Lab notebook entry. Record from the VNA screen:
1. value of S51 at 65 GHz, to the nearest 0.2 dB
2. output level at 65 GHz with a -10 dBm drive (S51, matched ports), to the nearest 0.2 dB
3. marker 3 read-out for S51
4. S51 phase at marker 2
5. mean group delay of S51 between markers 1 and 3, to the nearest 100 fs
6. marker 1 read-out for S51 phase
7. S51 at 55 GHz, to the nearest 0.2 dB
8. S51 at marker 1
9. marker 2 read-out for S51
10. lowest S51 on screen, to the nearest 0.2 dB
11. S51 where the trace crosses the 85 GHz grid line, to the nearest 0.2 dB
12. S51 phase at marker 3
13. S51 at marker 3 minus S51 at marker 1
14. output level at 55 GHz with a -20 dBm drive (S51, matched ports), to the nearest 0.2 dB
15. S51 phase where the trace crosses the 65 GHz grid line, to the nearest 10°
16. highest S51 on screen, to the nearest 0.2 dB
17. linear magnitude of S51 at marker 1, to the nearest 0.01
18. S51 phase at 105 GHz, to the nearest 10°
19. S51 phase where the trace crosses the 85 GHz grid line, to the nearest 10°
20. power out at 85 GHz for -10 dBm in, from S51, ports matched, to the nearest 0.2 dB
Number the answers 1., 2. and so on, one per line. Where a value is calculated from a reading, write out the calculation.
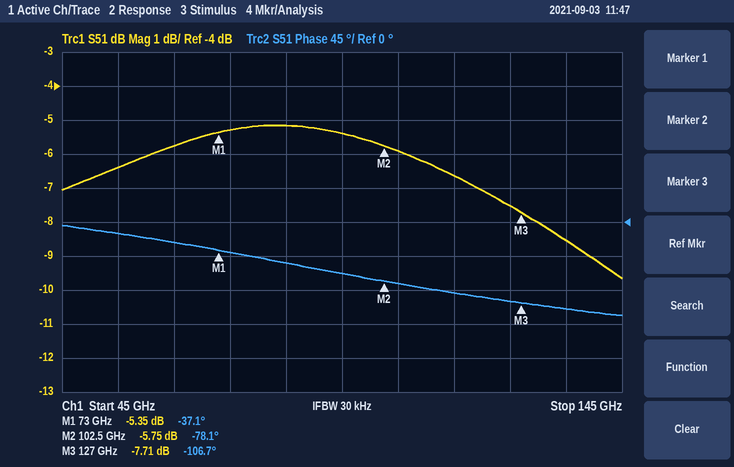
1. -5.8 dB
2. -10 dBm + (-5.8 dB) = -15.8 dBm
3. -7.71 dB
4. -78.1°
5. −(-106.7° − (-37.1°))/(360° × 54 GHz) ≈ 3.6 ps
6. -37.1°
7. -6.4 dB
8. -5.35 dB
9. -5.75 dB
10. -9.6 dB
11. -5.2 dB
12. -106.7°
13. -7.71 − (-5.35) = -2.36 dB
14. -20 dBm + (-6.4 dB) = -26.4 dBm
15. -30°
16. -5.2 dB
17. 10^(-5.35/20) ≈ 0.54
18. -80°
19. -50°
20. -10 dBm + (-5.2 dB) = -15.2 dBm
